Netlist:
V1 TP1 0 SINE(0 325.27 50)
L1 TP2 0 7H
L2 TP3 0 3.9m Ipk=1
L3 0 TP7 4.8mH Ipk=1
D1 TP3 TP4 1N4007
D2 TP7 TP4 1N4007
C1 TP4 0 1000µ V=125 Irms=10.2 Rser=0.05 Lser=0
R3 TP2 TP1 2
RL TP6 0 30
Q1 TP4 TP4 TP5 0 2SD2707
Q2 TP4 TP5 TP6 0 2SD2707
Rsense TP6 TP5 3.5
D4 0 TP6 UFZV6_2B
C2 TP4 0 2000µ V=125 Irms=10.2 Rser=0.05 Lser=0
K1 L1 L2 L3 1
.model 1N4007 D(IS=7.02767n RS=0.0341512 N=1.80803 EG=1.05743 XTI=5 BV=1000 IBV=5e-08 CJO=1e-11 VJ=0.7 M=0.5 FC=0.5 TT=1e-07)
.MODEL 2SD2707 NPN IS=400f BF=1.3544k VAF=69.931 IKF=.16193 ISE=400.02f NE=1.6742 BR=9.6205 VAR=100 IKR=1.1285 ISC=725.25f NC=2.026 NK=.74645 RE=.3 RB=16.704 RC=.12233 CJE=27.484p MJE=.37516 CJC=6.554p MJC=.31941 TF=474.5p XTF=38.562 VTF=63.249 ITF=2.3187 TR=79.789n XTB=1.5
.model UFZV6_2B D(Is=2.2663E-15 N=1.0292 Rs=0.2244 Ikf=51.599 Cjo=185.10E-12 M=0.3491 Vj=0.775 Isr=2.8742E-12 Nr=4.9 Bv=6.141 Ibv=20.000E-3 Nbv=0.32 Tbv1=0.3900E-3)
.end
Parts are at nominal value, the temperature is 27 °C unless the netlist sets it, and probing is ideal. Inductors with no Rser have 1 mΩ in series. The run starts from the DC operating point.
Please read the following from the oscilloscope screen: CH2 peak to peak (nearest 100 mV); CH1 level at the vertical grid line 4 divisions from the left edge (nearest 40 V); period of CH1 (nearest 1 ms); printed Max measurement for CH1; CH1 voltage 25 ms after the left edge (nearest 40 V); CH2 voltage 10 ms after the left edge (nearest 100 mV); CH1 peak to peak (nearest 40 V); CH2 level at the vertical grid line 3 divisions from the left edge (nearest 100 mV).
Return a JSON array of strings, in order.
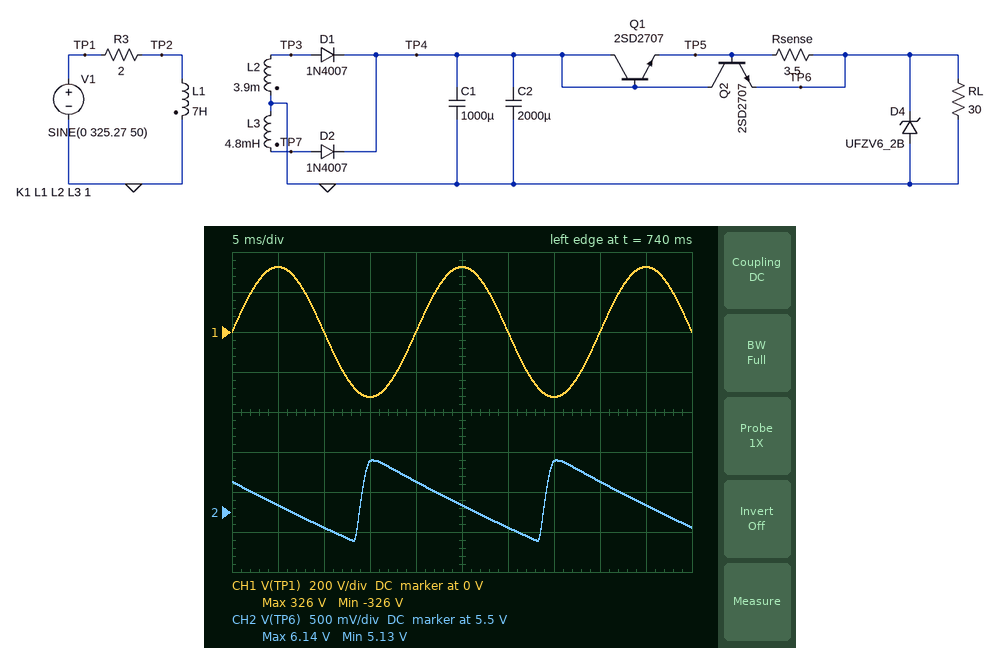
["1.0 V", "0 V", "20 ms", "326 V", "320 V", "5.3 V", "640 V", "6.1 V"]
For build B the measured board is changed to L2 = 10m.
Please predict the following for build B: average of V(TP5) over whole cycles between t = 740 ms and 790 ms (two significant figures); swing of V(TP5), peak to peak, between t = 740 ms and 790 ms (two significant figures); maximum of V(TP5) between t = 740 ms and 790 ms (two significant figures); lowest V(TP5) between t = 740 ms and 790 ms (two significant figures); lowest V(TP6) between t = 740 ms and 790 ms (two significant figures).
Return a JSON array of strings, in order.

["7.6 V", "2.1 V", "8.7 V", "6.6 V", "6.0 V"]
